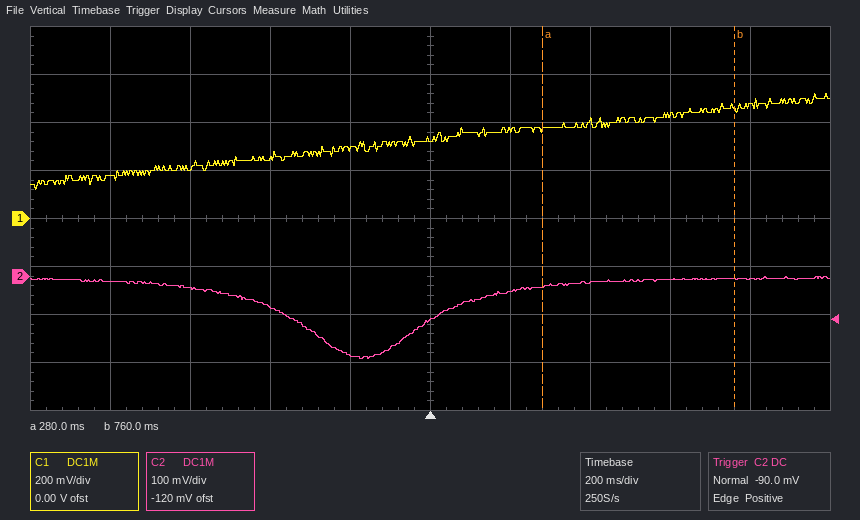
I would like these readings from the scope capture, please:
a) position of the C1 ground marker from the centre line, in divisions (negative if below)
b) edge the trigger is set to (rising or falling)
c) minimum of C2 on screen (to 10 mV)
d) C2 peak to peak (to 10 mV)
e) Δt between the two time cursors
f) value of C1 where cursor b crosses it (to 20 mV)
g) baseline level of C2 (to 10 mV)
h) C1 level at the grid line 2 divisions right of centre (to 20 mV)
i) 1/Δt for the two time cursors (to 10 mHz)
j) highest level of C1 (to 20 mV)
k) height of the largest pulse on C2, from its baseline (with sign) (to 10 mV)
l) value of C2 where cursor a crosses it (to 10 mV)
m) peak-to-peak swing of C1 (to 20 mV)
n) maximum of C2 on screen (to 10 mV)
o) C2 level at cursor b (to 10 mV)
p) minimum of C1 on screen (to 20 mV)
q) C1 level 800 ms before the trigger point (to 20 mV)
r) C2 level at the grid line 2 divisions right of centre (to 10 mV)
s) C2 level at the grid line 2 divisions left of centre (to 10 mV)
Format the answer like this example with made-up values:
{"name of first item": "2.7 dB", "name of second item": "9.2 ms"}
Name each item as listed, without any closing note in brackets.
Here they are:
{"position of the C1 ground marker from the centre line, in divisions": "0.0 div", "edge the trigger is set to": "rising", "minimum of C2 on screen": "-170 mV", "C2 peak to peak": "170 mV", "Δt between the two time cursors": "480 ms", "value of C1 where cursor b crosses it": "460 mV", "baseline level of C2": "-10 mV", "C1 level at the grid line 2 divisions right of centre": "400 mV", "1/Δt for the two time cursors": "2.08 Hz", "highest level of C1": "520 mV", "height of the largest pulse on C2, from its baseline (with sign)": "-160 mV", "value of C2 where cursor a crosses it": "-20 mV", "peak-to-peak swing of C1": "400 mV", "maximum of C2 on screen": "0 mV", "C2 level at cursor b": "-10 mV", "minimum of C1 on screen": "120 mV", "C1 level 800 ms before the trigger point": "180 mV", "C2 level at the grid line 2 divisions right of centre": "-10 mV", "C2 level at the grid line 2 divisions left of centre": "-60 mV"}
